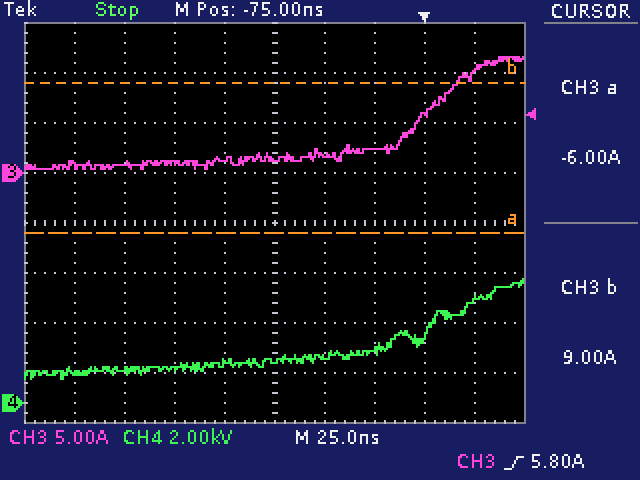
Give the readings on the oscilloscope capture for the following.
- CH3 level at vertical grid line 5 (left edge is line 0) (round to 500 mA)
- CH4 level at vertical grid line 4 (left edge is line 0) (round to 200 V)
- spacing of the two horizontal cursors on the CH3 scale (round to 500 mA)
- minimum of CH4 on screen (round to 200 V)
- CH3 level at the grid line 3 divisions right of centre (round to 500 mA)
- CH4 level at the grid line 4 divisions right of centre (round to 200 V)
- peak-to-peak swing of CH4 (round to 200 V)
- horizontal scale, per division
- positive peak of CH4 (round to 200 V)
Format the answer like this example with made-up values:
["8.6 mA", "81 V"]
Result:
["1.5 A", "1.6 kV", "15.0 A", "1.0 kV", "6.0 A", "4.2 kV", "4.0 kV", "25 ns", "5.0 kV"]
